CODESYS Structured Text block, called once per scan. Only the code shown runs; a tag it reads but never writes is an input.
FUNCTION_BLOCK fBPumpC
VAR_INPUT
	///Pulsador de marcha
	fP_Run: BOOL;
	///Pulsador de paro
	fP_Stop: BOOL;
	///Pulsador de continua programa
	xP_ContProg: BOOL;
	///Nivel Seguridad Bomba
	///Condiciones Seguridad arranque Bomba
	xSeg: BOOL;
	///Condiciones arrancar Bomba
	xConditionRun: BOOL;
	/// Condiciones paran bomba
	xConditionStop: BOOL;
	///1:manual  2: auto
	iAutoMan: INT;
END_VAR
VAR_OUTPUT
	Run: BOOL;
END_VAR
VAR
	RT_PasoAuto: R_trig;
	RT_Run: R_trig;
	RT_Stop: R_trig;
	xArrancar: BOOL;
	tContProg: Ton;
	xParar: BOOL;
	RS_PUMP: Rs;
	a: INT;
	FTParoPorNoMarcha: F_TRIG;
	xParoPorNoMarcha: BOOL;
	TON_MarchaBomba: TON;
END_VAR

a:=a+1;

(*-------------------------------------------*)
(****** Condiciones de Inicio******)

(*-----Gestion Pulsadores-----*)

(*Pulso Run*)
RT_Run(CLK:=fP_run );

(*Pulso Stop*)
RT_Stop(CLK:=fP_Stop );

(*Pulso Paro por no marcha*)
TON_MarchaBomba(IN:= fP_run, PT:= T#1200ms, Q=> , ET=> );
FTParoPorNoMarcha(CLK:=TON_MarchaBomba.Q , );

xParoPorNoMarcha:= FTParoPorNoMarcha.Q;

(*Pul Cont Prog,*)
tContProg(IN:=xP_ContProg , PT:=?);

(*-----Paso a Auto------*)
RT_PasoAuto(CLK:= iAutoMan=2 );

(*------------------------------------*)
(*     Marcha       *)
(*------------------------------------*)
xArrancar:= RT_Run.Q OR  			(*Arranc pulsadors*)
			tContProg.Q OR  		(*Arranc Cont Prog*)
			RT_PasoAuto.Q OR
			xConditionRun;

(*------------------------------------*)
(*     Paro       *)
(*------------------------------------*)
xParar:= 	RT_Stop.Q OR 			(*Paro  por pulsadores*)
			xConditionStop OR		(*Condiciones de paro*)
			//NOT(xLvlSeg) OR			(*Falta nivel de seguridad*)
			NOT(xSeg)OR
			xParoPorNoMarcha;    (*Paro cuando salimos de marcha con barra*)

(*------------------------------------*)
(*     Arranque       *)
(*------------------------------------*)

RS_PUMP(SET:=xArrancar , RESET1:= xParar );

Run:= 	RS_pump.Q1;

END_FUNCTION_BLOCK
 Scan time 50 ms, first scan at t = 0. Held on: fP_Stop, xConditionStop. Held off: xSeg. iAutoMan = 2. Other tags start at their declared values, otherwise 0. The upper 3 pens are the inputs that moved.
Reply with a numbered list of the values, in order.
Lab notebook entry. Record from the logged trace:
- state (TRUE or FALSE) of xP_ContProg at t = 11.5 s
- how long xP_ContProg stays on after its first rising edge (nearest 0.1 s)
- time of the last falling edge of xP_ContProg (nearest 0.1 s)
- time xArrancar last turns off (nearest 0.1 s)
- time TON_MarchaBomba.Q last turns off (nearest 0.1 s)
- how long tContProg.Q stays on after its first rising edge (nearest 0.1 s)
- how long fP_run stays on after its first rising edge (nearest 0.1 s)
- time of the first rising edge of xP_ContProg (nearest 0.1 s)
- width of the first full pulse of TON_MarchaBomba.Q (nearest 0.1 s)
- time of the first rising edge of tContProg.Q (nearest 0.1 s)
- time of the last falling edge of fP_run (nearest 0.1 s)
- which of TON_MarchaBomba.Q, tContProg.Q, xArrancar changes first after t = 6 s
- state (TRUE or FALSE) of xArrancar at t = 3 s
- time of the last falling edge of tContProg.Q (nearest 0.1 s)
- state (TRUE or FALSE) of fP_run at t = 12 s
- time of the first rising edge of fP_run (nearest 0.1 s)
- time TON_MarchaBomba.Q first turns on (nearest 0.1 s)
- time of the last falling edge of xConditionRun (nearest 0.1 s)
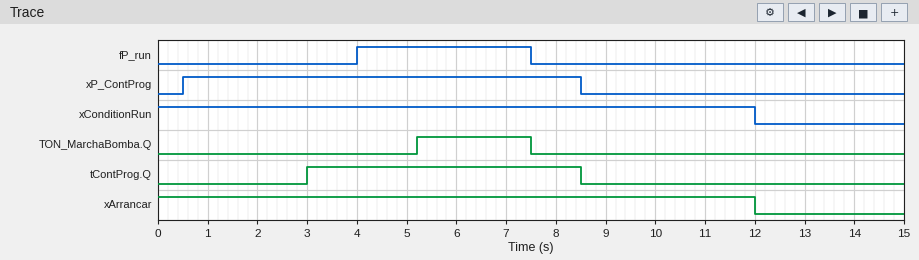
1. FALSE
2. 8.0 s
3. 8.5 s
4. 12.0 s
5. 7.5 s
6. 5.5 s
7. 3.5 s
8. 0.5 s
9. 2.3 s
10. 3.0 s
11. 7.5 s
12. TON_MarchaBomba.Q
13. TRUE
14. 8.5 s
15. FALSE
16. 4.0 s
17. 5.2 s
18. 12.0 s
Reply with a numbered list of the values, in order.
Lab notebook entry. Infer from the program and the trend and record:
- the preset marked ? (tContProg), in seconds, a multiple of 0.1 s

1. 2.5 s
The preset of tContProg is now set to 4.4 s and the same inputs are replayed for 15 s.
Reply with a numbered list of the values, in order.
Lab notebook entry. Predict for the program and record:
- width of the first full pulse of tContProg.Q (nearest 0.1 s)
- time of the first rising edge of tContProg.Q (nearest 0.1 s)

1. 3.6 s
2. 4.9 s
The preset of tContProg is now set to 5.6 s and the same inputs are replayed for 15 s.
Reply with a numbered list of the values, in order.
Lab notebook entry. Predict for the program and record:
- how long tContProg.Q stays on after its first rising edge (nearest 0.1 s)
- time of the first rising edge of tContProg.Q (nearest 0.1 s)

1. 2.4 s
2. 6.1 s
